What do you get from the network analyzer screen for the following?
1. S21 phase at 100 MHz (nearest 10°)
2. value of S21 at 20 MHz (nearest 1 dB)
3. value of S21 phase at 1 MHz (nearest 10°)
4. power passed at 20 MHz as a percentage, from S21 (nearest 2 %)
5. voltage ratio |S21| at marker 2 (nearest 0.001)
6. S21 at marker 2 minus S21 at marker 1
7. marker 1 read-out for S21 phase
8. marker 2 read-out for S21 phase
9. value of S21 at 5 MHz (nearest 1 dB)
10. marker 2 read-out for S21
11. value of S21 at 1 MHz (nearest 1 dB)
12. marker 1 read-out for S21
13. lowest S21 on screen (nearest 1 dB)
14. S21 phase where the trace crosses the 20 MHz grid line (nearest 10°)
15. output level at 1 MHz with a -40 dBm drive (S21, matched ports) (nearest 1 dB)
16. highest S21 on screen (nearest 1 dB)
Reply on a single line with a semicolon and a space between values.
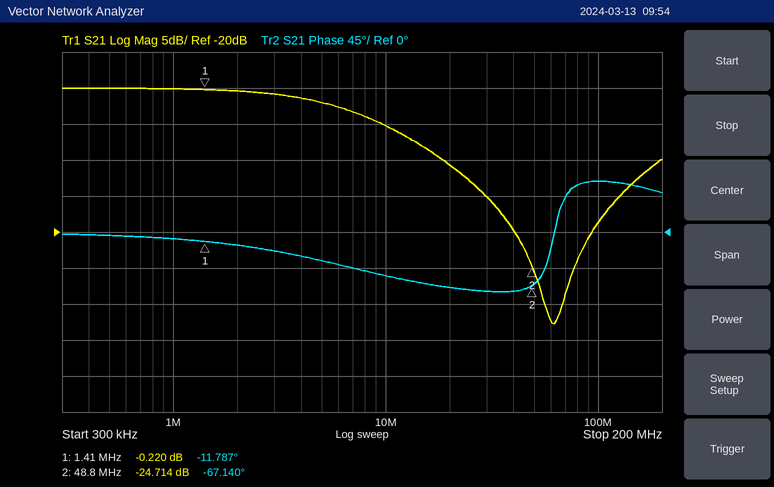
60°; -11 dB; -10°; 8 %; 0.058; -24.494 dB; -11.787°; -67.140°; -2 dB; -24.714 dB; 0 dB; -0.220 dB; -33 dB; -70°; -40 dBm; 0 dB
